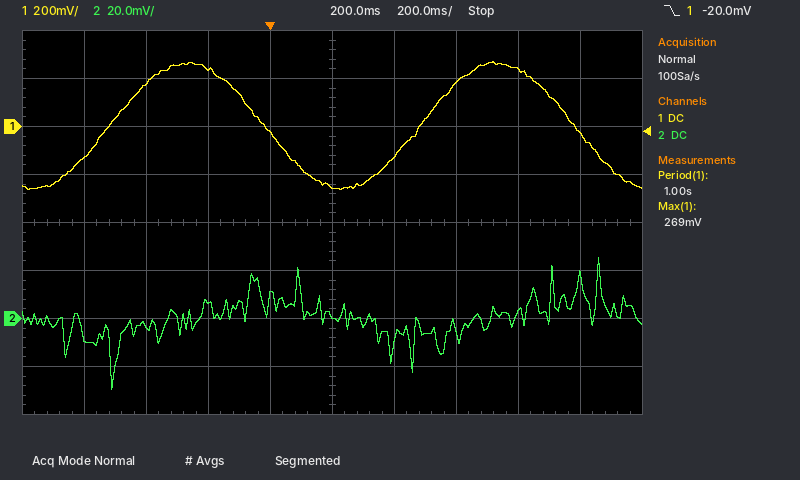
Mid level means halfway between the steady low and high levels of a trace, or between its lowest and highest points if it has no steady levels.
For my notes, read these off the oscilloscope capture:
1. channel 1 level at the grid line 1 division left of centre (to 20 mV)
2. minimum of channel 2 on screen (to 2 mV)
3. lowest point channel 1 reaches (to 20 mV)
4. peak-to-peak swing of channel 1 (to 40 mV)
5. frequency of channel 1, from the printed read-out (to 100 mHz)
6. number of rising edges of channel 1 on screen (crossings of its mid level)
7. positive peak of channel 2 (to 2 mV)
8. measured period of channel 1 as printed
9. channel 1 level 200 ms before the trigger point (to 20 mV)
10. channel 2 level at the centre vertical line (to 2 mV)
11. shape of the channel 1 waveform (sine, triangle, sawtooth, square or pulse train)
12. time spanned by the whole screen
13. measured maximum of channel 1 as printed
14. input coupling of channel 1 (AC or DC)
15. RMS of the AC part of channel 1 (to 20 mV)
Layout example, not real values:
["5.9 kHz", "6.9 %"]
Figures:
["-20 mV", "-30 mV", "-260 mV", "520 mV", "1.0 Hz", "2", "26 mV", "1.00 s", "240 mV", "2 mV", "sine", "2 s", "269 mV", "DC", "180 mV"]
